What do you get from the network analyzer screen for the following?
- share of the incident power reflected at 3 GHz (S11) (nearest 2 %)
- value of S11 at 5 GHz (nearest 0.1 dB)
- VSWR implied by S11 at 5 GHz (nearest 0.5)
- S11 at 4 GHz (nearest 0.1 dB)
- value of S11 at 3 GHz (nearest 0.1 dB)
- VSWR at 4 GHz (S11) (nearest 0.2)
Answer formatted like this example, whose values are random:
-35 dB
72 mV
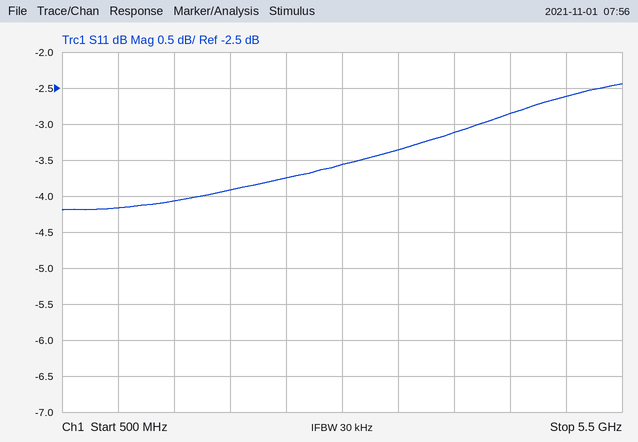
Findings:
44 %
-2.6 dB
6.5
-3.1 dB
-3.6 dB
5.6
